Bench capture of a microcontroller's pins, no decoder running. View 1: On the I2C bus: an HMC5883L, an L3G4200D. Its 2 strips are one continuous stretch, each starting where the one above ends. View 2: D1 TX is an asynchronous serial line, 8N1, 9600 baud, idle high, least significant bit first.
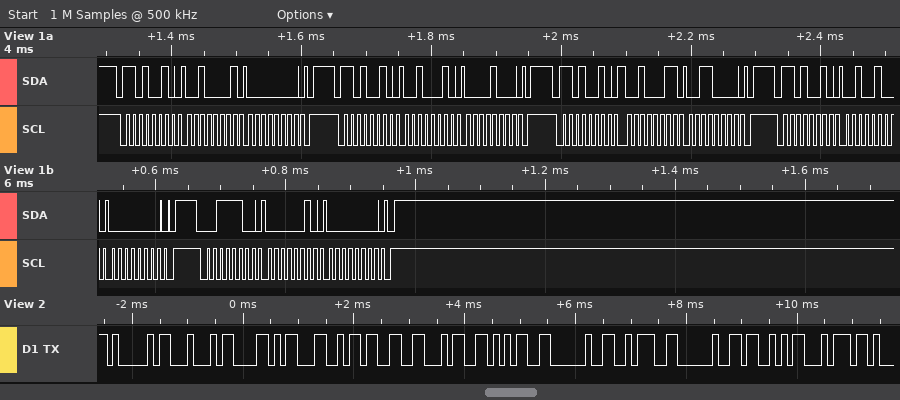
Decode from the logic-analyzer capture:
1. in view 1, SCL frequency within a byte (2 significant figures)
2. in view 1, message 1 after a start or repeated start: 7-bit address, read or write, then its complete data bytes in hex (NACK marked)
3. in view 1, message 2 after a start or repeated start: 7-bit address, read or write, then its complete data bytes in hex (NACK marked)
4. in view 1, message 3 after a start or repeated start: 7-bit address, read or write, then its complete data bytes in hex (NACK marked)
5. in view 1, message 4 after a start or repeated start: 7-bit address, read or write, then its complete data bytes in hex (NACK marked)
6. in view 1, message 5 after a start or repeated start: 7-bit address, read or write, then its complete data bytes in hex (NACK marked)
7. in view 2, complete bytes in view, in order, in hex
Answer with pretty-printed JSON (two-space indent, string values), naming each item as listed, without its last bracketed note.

{
  "in view 1, SCL frequency within a byte": "100 kHz",
  "in view 1, message 1 after a start or repeated start: 7-bit address, read or write, then its complete data bytes in hex": "0x69 write: 21 00",
  "in view 1, message 2 after a start or repeated start: 7-bit address, read or write, then its complete data bytes in hex": "0x69 write: 22 08",
  "in view 1, message 3 after a start or repeated start: 7-bit address, read or write, then its complete data bytes in hex": "0x69 write: 23 30",
  "in view 1, message 4 after a start or repeated start: 7-bit address, read or write, then its complete data bytes in hex": "0x69 write: 24 00",
  "in view 1, message 5 after a start or repeated start: 7-bit address, read or write, then its complete data bytes in hex": "0x1E write: 02 00",
  "in view 2, complete bytes in view, in order, in hex": "41 44 58 4C 33 34 35 20 3A 20 53 74"
}
